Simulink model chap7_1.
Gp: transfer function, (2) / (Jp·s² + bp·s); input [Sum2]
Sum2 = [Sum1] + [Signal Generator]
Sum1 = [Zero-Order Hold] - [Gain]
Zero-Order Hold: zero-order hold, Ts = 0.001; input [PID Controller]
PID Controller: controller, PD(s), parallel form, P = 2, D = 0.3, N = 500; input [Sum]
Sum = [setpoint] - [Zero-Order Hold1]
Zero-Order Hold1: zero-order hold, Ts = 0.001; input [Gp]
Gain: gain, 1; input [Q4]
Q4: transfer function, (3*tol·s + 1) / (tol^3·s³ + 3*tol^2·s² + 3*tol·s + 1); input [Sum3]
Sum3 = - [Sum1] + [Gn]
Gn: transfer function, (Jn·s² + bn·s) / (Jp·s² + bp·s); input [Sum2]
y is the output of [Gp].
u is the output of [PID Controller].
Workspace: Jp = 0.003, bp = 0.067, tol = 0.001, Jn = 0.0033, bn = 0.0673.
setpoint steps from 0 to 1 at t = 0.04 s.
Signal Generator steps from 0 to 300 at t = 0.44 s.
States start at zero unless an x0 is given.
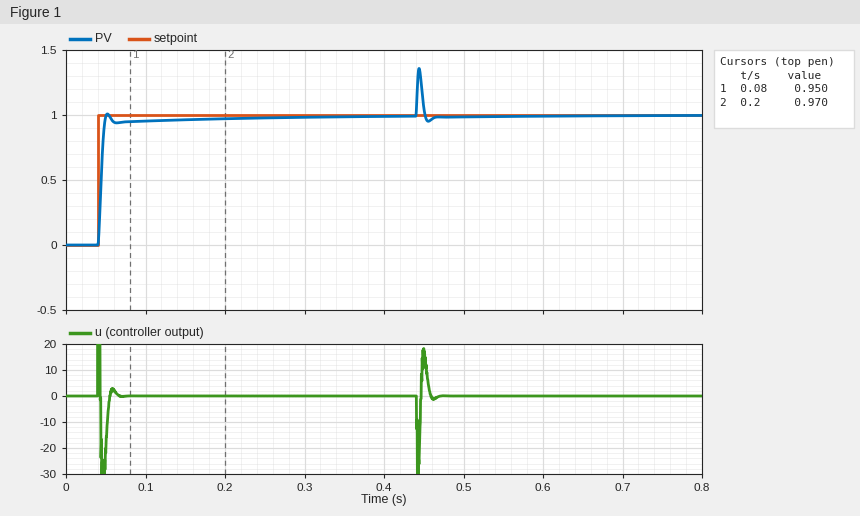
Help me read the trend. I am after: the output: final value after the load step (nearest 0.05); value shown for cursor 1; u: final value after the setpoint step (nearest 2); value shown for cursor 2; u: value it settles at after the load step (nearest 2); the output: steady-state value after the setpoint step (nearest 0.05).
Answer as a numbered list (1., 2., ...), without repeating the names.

1. 1.00
2. 0.950
3. 0
4. 0.970
5. 0
6. 1.00
